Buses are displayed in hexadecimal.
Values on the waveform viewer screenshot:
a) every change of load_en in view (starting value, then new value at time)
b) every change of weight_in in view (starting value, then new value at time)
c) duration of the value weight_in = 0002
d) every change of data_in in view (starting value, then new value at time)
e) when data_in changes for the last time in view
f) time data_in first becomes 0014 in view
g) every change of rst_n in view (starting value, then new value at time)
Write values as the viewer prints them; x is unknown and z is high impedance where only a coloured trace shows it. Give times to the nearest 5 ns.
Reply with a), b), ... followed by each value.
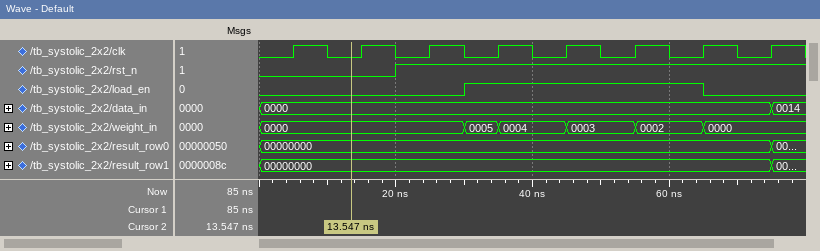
a) 0, 1 at 30 ns, 0 at 65 ns
b) 0000, 0005 at 30 ns, 0004 at 35 ns, 0003 at 45 ns, 0002 at 55 ns, 0000 at 65 ns
c) 10 ns
d) 0000, 0014 at 75 ns
e) 75 ns
f) 75 ns
g) 0, 1 at 20 ns
